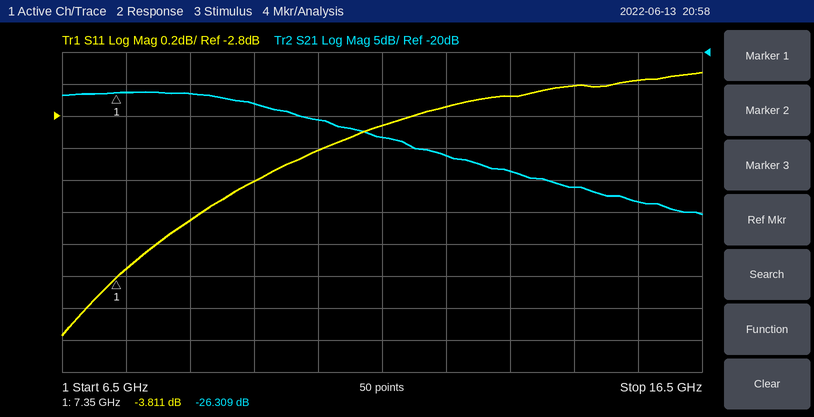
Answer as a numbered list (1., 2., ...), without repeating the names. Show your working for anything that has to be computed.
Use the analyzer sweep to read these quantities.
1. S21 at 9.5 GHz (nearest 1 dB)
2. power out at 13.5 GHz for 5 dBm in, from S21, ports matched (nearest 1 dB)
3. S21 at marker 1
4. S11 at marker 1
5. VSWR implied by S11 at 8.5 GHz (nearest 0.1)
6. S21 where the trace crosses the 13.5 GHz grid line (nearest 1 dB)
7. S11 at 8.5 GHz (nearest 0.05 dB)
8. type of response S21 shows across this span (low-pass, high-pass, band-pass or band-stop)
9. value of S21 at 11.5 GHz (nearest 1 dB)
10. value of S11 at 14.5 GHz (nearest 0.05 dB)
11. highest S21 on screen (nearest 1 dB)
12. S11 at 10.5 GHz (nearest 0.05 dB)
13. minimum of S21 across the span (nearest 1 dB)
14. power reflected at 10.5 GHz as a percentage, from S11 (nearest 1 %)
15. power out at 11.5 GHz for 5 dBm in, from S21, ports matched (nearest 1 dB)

1. -28 dB
2. 5 dBm + (-39 dB) = -34 dBm
3. -26.309 dB
4. -3.811 dB
5. |Γ| = 10^(-3.45/20) = 0.6722; VSWR = (1 + 0.6722)/(1 − 0.6722) ≈ 5.1
6. -39 dB
7. -3.45 dB
8. low-pass
9. -33 dB
10. -2.60 dB
11. -26 dB
12. -3.00 dB
13. -45 dB
14. 10^(-3/10) ≈ 50 %
15. 5 dBm + (-33 dB) = -28 dBm
